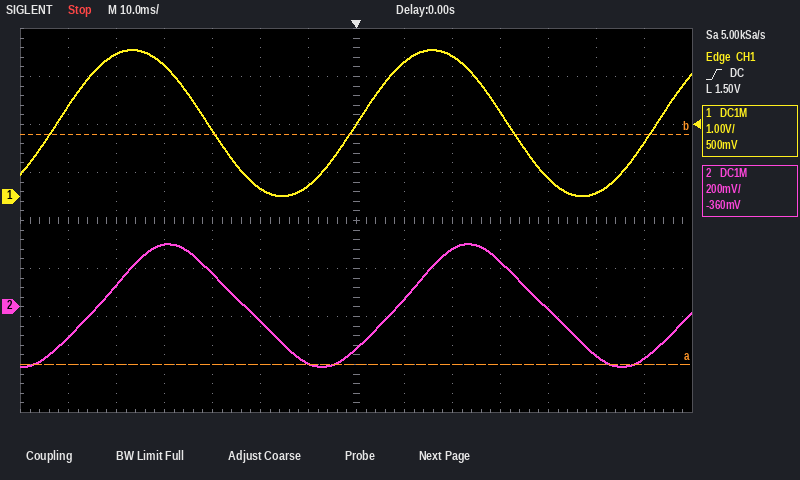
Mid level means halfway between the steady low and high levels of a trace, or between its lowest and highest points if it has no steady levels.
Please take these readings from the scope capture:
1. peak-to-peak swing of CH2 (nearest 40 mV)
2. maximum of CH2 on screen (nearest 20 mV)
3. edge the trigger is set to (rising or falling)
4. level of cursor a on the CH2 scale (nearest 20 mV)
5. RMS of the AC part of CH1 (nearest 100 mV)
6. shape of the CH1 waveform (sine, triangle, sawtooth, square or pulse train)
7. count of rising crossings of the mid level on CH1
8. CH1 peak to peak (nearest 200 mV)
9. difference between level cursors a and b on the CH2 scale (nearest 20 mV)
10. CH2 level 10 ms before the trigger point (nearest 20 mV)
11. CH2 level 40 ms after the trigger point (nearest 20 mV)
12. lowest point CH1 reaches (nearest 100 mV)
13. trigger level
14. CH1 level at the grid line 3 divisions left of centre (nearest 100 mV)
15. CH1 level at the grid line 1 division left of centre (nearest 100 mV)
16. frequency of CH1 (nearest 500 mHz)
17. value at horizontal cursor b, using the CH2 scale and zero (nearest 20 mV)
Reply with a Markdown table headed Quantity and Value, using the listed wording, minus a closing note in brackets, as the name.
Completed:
| Quantity | Value |
|---|---|
| peak-to-peak swing of CH2 | 520 mV |
| maximum of CH2 on screen | 260 mV |
| edge the trigger is set to | rising |
| level of cursor a on the CH2 scale | -240 mV |
| RMS of the AC part of CH1 | 1.1 V |
| shape of the CH1 waveform | sine |
| count of rising crossings of the mid level on CH1 | 3 |
| CH1 peak to peak | 3.0 V |
| difference between level cursors a and b on the CH2 scale | 960 mV |
| CH2 level 10 ms before the trigger point | -240 mV |
| CH2 level 40 ms after the trigger point | 0 mV |
| lowest point CH1 reaches | 0.0 V |
| trigger level | 1.50 V |
| CH1 level at the grid line 3 divisions left of centre | 1.4 V |
| CH1 level at the grid line 1 division left of centre | 200 mV |
| frequency of CH1 | 16.0 Hz |
| value at horizontal cursor b, using the CH2 scale and zero | 720 mV |
